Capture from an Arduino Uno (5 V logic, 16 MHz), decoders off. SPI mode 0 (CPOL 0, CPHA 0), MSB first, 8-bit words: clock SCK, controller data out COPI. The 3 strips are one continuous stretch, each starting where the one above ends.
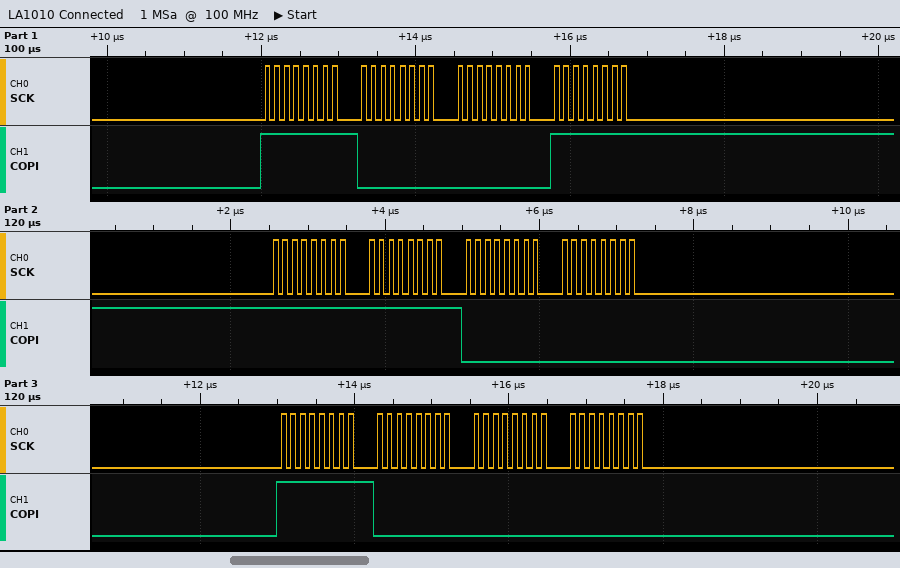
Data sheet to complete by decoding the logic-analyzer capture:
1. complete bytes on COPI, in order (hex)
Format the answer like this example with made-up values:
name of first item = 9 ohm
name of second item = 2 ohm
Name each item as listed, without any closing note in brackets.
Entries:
complete bytes on COPI, in order = FF 00 00 FF FF FF 00 00 FF 00 00 00
